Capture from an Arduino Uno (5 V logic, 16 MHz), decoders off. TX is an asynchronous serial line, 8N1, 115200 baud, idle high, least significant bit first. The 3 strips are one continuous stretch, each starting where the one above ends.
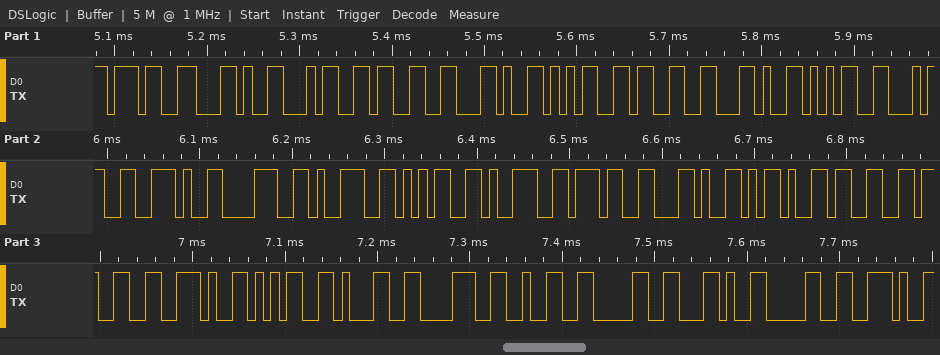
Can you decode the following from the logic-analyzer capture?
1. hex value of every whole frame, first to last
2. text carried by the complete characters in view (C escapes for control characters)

37 2C 34 33 2C 35 33 2C 35 34 2E 38 39 35 39 37 2C 2D 33 33 2E 35 31 38 32 30 2C 30 2E
"7,43,53,54.89597,-33.51820,0."
